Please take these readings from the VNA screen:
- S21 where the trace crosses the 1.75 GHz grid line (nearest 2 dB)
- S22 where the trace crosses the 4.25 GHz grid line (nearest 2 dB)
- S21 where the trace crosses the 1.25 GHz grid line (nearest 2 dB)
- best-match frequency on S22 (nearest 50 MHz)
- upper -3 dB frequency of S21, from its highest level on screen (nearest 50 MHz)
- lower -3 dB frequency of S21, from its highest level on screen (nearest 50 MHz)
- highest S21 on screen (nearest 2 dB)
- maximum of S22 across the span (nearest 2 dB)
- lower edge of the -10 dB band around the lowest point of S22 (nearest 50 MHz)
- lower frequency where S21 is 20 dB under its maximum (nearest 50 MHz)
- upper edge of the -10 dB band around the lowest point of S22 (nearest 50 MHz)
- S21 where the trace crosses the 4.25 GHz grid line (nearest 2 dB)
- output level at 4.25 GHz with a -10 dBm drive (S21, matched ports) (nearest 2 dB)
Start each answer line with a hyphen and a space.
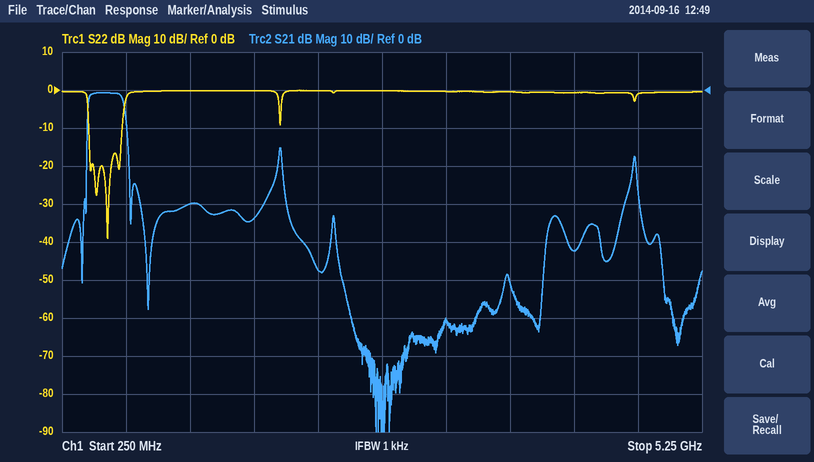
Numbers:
- -34 dB
- 0 dB
- -30 dB
- 600 MHz
- 750 MHz
- 450 MHz
- 0 dB
- 0 dB
- 450 MHz
- 450 MHz
- 700 MHz
- -42 dB
- -52 dBm
